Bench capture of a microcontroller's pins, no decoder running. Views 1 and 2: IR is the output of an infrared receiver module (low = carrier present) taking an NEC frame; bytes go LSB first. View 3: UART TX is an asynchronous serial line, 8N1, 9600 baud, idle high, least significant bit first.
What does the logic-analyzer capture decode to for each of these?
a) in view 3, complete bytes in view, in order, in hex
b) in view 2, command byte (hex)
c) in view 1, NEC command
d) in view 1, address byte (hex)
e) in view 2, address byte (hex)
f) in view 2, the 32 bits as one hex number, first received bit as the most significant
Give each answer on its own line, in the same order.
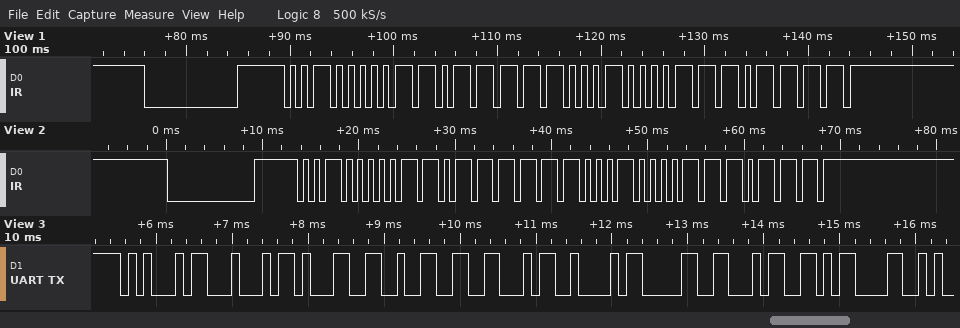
0x45 0x44 0x31 0x32 0x46 0x42 0x30 0x34 0x0D
0x11
0x08
0x04
0x04
0x20DF8877
